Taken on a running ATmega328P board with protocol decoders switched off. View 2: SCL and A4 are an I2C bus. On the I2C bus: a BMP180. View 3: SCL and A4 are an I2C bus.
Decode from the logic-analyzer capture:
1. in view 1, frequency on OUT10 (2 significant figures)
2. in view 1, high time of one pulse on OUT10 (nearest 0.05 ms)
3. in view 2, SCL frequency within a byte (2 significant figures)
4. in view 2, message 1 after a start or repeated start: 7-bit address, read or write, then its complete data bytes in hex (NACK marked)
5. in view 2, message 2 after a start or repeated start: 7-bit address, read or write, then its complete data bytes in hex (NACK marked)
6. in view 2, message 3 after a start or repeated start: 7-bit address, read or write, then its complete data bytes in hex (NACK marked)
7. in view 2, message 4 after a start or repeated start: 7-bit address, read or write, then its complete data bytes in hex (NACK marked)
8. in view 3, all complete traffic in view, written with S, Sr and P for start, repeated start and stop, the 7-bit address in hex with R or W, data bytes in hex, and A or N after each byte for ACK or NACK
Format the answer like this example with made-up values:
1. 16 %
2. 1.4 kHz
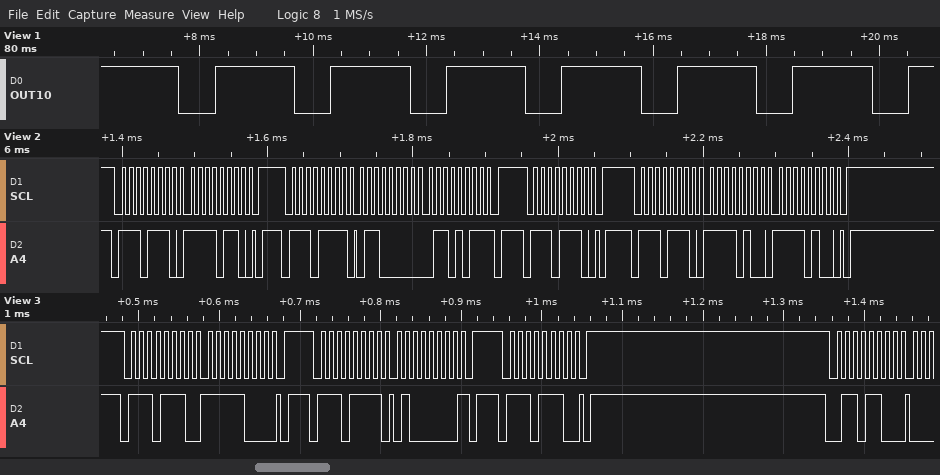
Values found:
1. 490 Hz
2. 1.40 ms
3. 100 kHz
4. 0x77 write: F6
5. 0x77 read: 60 6B NACK
6. 0x77 write
7. 0x77 write: F4 F4
8. S 77W A F8 A P S 77R A 40 N P S 77W A P S 36W A
